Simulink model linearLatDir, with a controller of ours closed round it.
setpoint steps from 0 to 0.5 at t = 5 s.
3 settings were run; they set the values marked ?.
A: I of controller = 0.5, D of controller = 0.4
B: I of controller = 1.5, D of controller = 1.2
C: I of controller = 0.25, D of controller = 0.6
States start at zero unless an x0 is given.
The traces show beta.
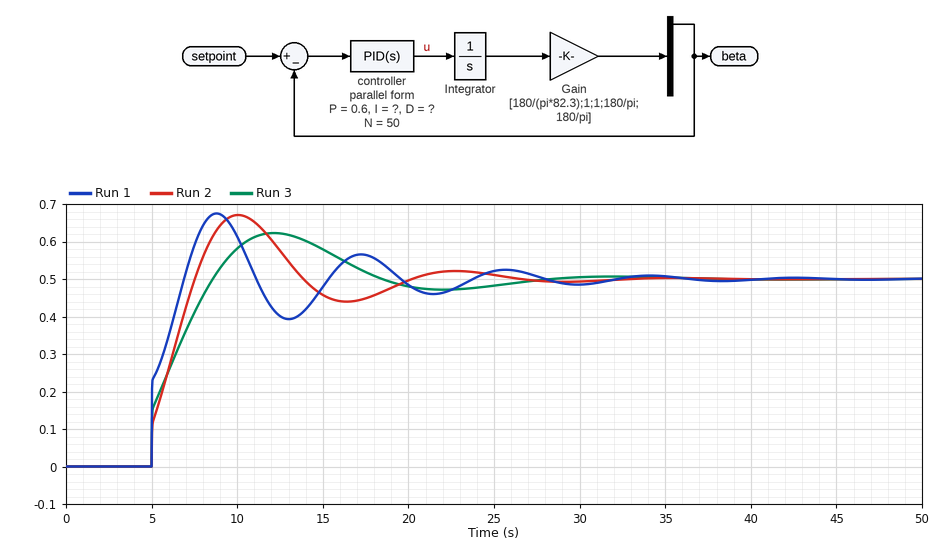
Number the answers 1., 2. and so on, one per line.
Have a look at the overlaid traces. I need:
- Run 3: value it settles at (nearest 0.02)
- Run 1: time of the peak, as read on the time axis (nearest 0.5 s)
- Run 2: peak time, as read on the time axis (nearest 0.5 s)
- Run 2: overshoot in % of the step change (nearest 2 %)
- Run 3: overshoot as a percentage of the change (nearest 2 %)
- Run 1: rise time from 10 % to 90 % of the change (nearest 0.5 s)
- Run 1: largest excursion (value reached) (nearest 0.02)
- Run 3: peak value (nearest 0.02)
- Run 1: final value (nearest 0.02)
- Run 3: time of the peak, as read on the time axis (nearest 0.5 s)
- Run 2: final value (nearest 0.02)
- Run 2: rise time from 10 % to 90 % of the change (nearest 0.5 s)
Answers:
1. 0.50
2. 9.0 s
3. 10.0 s
4. 34 %
5. 24 %
6. 1.5 s
7. 0.68
8. 0.62
9. 0.50
10. 12.0 s
11. 0.50
12. 2.0 s
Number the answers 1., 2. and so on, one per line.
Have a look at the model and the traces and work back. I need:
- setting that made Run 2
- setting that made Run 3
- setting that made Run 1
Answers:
1. A
2. C
3. B
